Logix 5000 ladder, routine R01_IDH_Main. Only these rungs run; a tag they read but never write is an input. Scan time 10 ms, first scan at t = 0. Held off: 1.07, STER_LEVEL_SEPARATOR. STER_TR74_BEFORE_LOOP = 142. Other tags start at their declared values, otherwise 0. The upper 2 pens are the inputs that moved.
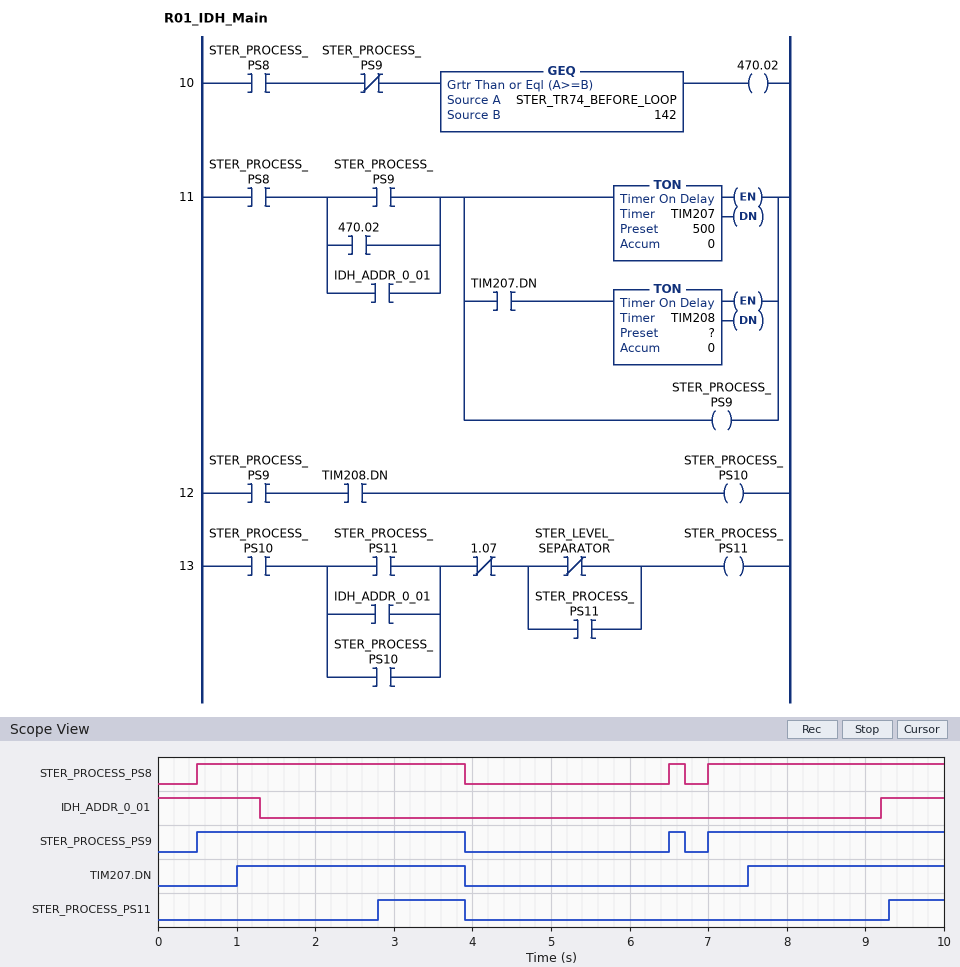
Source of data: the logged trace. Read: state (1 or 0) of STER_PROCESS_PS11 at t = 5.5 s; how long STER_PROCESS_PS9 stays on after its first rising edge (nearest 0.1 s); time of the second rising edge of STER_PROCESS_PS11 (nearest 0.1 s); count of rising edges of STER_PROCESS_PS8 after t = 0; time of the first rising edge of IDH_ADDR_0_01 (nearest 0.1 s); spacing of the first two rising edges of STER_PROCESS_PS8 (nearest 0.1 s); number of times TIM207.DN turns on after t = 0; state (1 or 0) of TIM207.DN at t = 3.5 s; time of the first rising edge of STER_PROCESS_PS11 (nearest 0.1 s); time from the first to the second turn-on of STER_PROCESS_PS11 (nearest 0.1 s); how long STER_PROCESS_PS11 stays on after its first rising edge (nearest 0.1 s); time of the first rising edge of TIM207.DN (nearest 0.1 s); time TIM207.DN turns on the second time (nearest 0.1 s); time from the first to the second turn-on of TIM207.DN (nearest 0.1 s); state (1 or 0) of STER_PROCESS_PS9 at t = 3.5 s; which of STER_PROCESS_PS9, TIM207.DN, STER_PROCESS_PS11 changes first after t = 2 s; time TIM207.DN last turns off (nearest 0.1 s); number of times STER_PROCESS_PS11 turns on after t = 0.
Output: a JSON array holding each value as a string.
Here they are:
["0", "3.4 s", "9.3 s", "3", "9.2 s", "6.0 s", "2", "1", "2.8 s", "6.5 s", "1.1 s", "1.0 s", "7.5 s", "6.5 s", "1", "STER_PROCESS_PS11", "3.9 s", "2"]
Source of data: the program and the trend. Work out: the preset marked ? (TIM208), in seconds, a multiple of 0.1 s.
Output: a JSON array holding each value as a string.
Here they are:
["1.8 s"]
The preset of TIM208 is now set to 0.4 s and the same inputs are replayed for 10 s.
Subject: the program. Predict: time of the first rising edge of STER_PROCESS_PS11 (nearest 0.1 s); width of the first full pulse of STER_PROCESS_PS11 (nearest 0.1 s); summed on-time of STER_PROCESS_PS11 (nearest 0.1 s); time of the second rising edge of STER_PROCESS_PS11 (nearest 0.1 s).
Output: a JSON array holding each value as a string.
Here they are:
["1.4 s", "2.5 s", "4.6 s", "7.9 s"]
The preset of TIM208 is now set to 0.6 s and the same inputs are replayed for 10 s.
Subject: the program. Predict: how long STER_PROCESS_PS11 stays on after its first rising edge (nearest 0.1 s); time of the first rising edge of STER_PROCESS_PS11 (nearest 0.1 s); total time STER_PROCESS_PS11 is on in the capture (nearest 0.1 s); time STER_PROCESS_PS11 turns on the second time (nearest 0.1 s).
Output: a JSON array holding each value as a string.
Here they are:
["2.3 s", "1.6 s", "4.2 s", "8.1 s"]
